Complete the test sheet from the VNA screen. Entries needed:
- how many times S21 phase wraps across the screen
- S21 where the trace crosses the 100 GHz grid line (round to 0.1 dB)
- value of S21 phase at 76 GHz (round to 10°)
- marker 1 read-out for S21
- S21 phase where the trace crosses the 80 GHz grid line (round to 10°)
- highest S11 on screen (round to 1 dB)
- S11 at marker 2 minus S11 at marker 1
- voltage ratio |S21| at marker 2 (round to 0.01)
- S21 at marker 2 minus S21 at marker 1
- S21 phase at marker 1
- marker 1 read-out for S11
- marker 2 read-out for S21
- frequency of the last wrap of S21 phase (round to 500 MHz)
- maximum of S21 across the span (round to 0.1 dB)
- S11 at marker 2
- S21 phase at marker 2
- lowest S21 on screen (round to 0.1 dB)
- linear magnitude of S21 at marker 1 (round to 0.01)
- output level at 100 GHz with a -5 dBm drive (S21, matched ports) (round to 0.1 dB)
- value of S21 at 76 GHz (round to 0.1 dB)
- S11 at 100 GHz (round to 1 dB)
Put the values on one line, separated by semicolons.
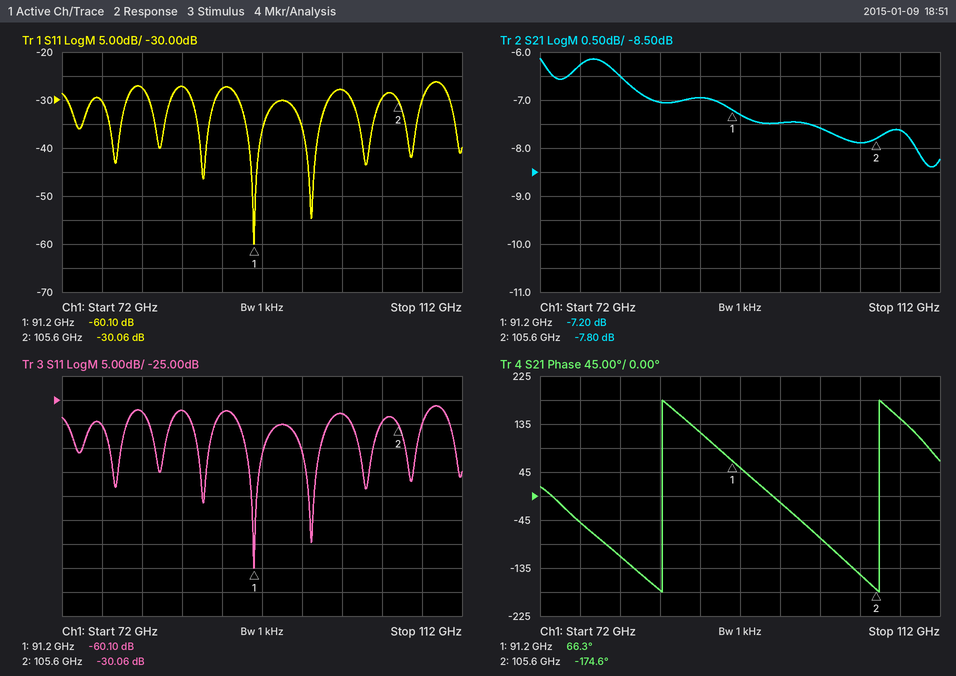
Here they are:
2; -7.6 dB; -50°; -7.20 dB; -110°; -26 dB; 30.04 dB; 0.41; -0.60 dB; 66.3°; -60.10 dB; -7.80 dB; 106.0 GHz; -6.1 dB; -30.06 dB; -174.6°; -8.4 dB; 0.44; -12.6 dBm; -6.3 dB; -28 dB
